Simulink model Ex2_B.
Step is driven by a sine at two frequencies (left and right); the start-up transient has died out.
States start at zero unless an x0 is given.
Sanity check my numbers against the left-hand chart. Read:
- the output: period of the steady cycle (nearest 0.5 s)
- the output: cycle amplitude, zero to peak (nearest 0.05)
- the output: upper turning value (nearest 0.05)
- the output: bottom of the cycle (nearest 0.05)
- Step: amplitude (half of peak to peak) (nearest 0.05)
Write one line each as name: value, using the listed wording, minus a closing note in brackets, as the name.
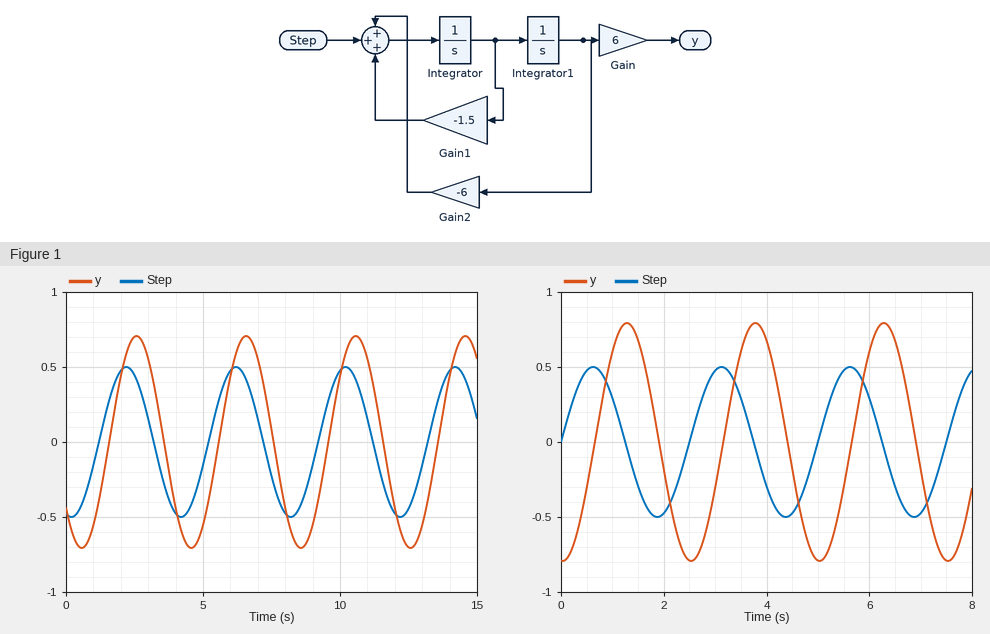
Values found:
the output: period of the steady cycle: 4.0 s
the output: cycle amplitude, zero to peak: 0.70
the output: upper turning value: 0.70
the output: bottom of the cycle: -0.70
Step: amplitude (half of peak to peak): 0.50
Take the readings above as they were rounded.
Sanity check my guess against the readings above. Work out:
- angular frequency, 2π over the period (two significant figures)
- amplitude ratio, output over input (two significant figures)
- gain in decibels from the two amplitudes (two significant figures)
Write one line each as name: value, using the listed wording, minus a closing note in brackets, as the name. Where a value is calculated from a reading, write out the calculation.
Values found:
angular frequency, 2π over the period: 2π / 4 = 1.6 rad/s
amplitude ratio, output over input: 0.7 / 0.5 = 1.4
gain in decibels from the two amplitudes: 20 log10(0.7 / 0.5) = 2.9 dB
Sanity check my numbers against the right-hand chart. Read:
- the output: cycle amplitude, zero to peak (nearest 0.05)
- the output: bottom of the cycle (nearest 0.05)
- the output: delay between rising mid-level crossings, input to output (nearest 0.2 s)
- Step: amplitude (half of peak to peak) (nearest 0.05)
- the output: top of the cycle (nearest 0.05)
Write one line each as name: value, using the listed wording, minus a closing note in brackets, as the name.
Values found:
the output: cycle amplitude, zero to peak: 0.80
the output: bottom of the cycle: -0.80
the output: delay between rising mid-level crossings, input to output: 0.6 s
Step: amplitude (half of peak to peak): 0.50
the output: top of the cycle: 0.80
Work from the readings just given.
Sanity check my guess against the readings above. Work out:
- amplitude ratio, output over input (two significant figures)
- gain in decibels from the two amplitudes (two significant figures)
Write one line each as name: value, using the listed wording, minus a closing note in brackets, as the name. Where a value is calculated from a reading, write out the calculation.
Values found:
amplitude ratio, output over input: 0.8 / 0.5 = 1.6
gain in decibels from the two amplitudes: 20 log10(0.8 / 0.5) = 4.1 dB
